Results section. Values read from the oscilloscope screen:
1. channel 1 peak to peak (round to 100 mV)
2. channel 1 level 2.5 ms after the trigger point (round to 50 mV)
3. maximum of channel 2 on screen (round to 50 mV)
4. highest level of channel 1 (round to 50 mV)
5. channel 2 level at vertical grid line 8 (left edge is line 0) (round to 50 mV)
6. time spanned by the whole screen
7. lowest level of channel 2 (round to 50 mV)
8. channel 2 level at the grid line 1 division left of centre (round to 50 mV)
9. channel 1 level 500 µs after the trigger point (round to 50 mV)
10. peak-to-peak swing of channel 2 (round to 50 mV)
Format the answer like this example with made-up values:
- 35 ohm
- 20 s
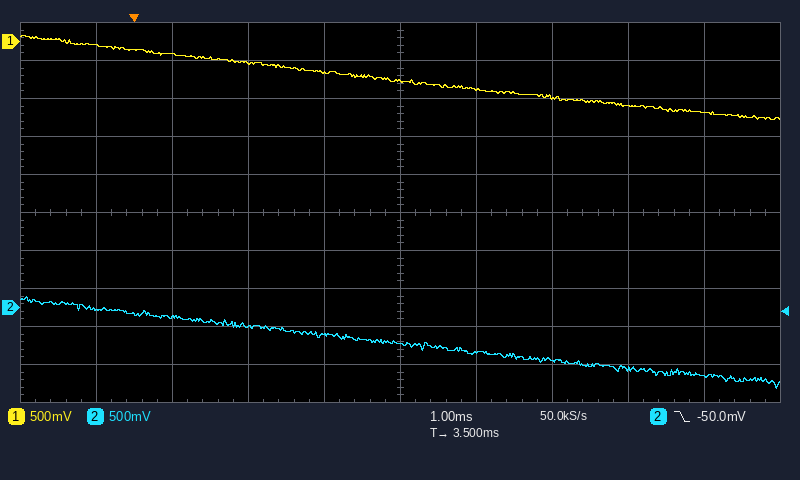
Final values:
- 1.10 V
- -400 mV
- 150 mV
- 100 mV
- -800 mV
- 10 ms
- -1.05 V
- -350 mV
- -150 mV
- 1.20 V
